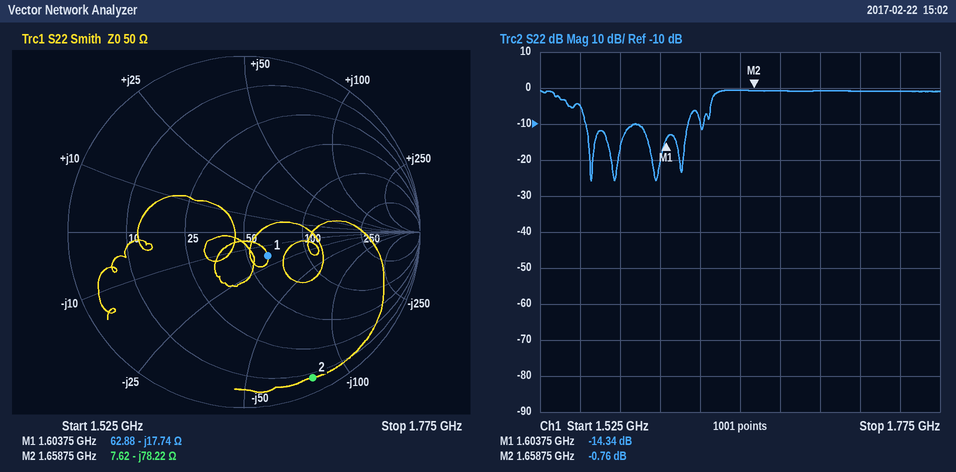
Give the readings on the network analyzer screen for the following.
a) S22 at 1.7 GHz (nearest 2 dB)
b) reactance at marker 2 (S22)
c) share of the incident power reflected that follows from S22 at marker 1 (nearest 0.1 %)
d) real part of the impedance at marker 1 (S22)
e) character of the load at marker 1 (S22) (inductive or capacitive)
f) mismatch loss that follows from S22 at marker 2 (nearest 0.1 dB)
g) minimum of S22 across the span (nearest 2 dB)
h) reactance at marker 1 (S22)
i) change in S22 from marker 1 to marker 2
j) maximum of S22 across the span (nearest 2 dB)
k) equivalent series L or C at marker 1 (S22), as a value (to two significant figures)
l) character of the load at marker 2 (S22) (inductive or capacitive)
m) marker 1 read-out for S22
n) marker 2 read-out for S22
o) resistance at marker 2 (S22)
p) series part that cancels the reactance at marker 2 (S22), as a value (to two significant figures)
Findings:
0 dB
-78.22 Ω
3.7 %
62.88 Ω
capacitive
7.9 dB
-26 dB
-17.74 Ω
13.58 dB
0 dB
5.6 pF
capacitive
-14.34 dB
-0.76 dB
7.62 Ω
7.5 nH
